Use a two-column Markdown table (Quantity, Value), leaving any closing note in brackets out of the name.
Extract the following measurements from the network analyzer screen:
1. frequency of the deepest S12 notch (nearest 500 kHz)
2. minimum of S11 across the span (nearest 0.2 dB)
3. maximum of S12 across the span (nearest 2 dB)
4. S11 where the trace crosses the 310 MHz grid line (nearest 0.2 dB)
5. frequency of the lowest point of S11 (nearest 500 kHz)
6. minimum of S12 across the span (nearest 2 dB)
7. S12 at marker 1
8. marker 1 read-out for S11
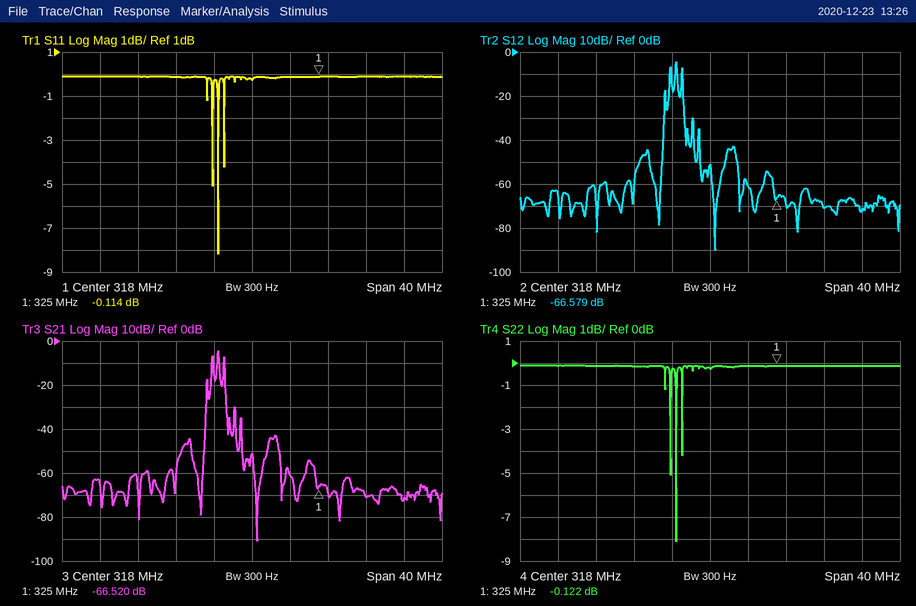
| Quantity | Value |
|---|---|
| frequency of the deepest S12 notch | 318.5 MHz |
| minimum of S11 across the span | -8.2 dB |
| maximum of S12 across the span | -4 dB |
| S11 where the trace crosses the 310 MHz grid line | -0.2 dB |
| frequency of the lowest point of S11 | 314.5 MHz |
| minimum of S12 across the span | -90 dB |
| S12 at marker 1 | -66.579 dB |
| marker 1 read-out for S11 | -0.114 dB |
